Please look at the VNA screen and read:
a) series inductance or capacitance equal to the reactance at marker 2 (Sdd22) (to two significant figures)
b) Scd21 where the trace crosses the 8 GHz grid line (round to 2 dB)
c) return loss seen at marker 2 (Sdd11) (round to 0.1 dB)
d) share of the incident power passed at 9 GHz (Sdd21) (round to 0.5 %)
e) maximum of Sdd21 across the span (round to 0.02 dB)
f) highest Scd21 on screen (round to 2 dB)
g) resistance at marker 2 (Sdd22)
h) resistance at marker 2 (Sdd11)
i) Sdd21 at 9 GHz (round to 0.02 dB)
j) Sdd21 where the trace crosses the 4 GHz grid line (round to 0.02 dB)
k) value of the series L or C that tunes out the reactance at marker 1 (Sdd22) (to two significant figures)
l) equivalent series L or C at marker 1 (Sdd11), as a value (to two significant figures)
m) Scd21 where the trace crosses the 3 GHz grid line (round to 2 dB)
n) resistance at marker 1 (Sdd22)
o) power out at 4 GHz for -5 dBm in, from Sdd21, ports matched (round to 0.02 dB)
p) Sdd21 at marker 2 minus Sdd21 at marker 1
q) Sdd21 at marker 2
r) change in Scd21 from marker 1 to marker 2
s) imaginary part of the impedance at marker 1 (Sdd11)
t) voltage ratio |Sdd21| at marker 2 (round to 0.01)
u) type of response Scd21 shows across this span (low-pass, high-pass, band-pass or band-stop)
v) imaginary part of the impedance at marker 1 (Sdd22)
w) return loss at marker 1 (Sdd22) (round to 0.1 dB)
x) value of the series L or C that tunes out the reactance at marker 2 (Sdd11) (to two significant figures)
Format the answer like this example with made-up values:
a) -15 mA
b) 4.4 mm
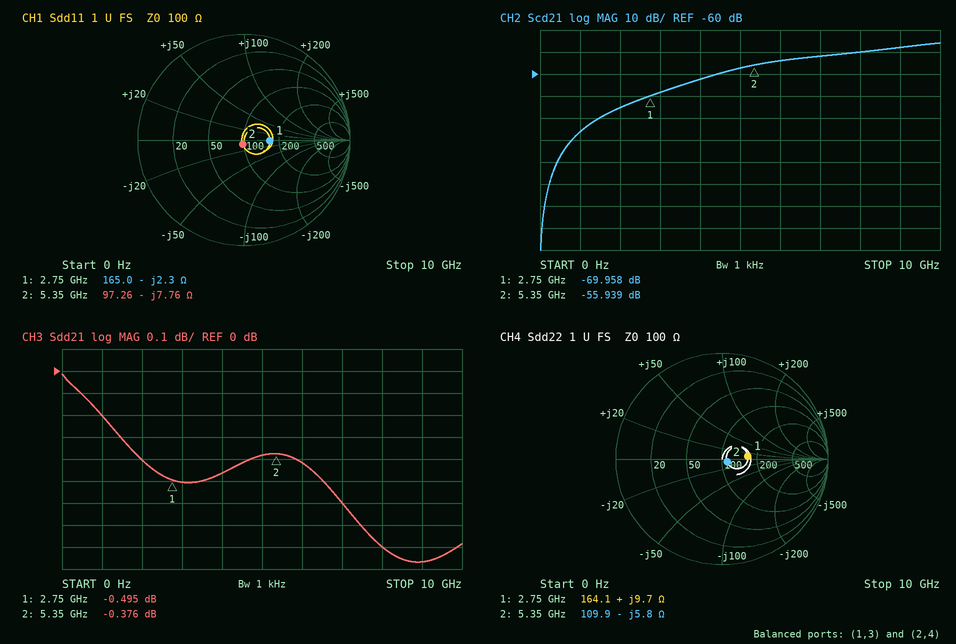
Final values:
a) 5.1 pF
b) -50 dB
c) 27.6 dB
d) 82.0 %
e) -0.02 dB
f) -46 dB
g) 109.9 Ω
h) 97.26 Ω
i) -0.86 dB
j) -0.46 dB
k) 6.0 pF
l) 25 pF
m) -68 dB
n) 164.1 Ω
o) -5.46 dBm
p) 0.119 dB
q) -0.376 dB
r) 14.019 dB
s) -2.3 Ω
t) 0.96
u) high-pass
v) +9.7 Ω
w) 12.2 dB
x) 230 pH
